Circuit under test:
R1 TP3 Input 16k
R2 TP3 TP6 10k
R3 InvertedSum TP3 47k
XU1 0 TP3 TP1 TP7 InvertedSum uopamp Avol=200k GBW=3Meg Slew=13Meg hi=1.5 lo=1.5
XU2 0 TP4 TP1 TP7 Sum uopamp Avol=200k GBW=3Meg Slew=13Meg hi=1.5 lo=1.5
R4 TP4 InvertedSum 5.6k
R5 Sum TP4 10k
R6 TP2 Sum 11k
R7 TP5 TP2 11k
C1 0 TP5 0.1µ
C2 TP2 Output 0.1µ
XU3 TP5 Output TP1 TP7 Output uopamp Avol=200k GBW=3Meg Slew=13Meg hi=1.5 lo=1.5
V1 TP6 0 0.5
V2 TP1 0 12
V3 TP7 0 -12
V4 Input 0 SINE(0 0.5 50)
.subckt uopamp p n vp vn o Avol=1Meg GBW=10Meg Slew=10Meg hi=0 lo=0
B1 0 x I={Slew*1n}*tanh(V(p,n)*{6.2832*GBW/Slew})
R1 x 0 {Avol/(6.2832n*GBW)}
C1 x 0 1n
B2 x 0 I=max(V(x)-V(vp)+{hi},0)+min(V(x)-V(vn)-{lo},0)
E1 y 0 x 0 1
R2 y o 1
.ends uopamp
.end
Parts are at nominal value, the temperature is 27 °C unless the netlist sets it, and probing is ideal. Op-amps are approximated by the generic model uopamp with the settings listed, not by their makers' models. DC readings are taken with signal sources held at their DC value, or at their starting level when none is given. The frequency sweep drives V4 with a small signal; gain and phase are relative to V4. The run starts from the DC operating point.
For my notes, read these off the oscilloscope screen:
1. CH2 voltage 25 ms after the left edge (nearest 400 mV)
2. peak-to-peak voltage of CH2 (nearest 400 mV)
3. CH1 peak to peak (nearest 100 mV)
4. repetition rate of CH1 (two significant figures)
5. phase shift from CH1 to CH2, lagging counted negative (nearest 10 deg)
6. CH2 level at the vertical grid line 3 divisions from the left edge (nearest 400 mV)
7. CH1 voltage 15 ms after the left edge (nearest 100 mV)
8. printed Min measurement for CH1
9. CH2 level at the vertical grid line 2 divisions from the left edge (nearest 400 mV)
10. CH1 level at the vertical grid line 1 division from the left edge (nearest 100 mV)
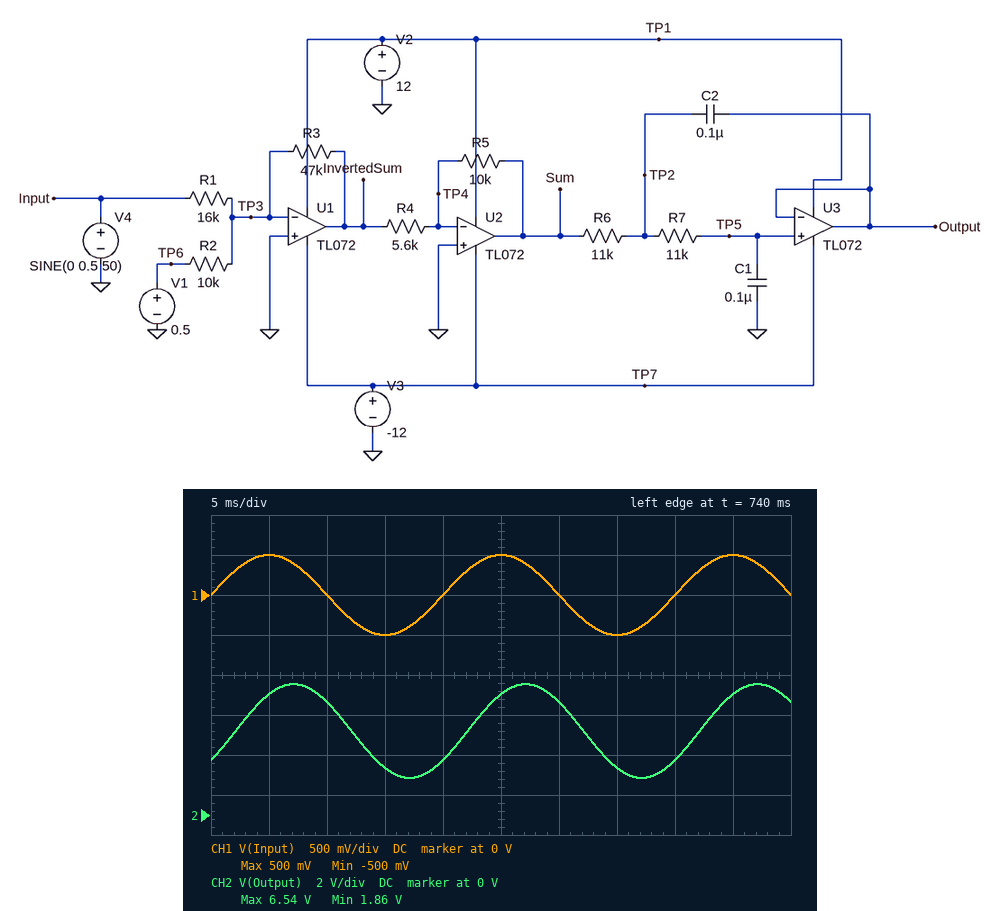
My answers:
6.0 V
4.8 V
1.0 V
50 Hz
-40 deg
2.4 V
-500 mV
-500 mV
5.6 V
500 mV
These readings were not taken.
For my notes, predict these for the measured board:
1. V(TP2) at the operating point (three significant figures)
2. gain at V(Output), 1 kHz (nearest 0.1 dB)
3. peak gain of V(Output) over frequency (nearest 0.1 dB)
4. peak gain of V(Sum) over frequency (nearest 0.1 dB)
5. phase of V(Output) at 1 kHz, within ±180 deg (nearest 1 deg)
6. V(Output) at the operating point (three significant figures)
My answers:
4.20 V
-19.4 dB
14.4 dB
14.4 dB
-164 deg
4.20 V
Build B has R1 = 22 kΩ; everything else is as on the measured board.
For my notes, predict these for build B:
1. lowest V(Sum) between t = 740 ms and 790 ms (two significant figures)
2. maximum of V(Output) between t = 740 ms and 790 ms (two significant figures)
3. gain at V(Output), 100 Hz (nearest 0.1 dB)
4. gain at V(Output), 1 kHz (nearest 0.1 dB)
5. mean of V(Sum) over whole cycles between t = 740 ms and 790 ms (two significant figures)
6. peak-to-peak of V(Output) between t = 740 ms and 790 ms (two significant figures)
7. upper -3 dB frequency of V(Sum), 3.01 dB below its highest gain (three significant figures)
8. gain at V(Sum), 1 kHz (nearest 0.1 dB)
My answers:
2.3 V
5.9 V
8.2 dB
-22.1 dB
4.2 V
3.4 V
345 kHz
11.6 dB
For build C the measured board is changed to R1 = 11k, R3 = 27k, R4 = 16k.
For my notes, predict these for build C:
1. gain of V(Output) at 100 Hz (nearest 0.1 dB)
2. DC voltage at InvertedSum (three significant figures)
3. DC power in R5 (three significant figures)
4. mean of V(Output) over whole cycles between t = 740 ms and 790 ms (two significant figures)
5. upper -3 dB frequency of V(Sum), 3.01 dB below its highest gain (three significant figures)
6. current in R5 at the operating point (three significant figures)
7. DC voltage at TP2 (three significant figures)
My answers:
0.3 dB
-1.35 V
71.2 µW
840 mV
458 kHz
84.4 µA
844 mV
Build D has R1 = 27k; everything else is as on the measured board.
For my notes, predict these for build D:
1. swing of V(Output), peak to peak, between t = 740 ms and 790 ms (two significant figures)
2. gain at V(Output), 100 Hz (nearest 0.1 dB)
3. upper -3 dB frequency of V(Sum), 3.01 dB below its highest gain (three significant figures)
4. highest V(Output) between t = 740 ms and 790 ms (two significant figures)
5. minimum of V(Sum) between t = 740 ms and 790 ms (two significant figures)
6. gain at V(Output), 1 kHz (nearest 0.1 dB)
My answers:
2.8 V
6.5 dB
360 kHz
5.6 V
2.6 V
-23.9 dB
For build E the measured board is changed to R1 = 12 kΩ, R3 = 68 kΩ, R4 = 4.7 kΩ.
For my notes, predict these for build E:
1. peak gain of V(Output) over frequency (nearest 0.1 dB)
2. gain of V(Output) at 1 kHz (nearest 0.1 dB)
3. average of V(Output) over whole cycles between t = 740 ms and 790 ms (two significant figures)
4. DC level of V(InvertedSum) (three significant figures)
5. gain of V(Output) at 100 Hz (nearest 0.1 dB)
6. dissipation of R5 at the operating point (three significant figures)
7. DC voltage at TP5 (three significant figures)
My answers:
21.6 dB
-12.1 dB
6.7 V
-3.40 V
18.2 dB
5.23 mW
7.23 V
